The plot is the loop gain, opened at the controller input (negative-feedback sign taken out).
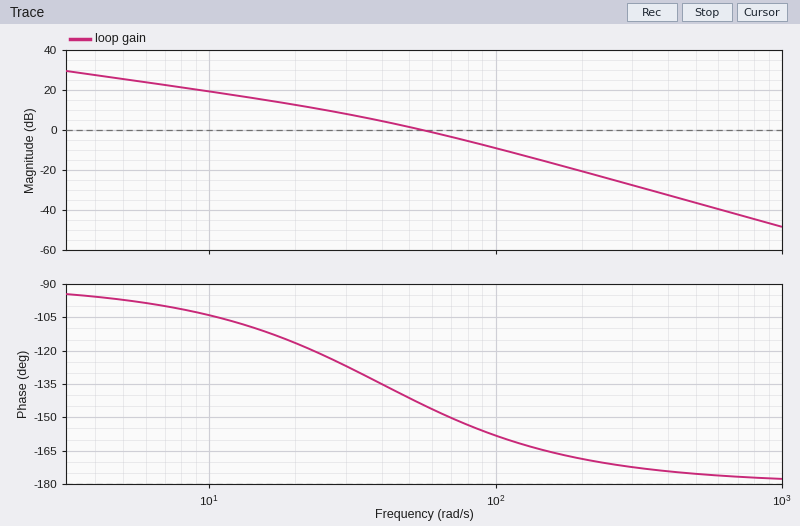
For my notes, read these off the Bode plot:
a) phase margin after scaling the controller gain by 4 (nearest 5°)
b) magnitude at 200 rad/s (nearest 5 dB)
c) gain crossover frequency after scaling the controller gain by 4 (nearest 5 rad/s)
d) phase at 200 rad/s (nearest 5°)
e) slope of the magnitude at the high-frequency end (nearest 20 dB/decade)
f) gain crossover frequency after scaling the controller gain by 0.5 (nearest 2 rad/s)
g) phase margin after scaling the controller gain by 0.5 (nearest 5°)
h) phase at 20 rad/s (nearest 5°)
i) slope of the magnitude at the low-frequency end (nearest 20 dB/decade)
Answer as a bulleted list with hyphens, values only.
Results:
- 20°
- -20 dB
- 120 rad/s
- -170°
- -40 dB/decade
- 36 rad/s
- 50°
- -115°
- -20 dB/decade
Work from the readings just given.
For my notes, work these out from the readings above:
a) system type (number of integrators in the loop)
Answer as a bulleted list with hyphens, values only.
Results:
- 1
